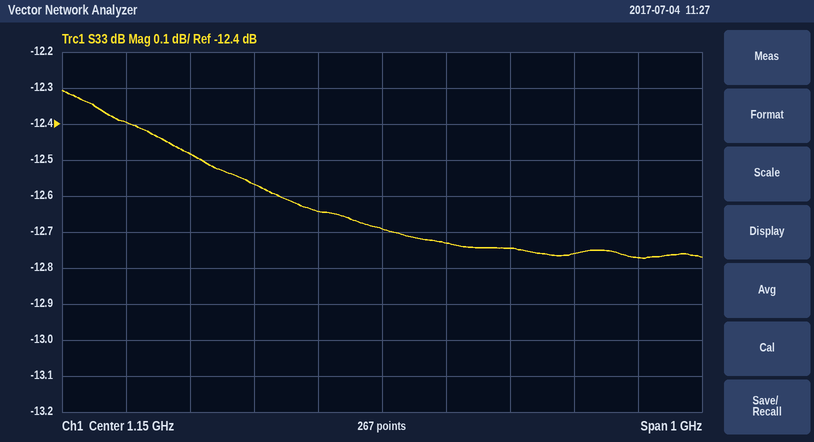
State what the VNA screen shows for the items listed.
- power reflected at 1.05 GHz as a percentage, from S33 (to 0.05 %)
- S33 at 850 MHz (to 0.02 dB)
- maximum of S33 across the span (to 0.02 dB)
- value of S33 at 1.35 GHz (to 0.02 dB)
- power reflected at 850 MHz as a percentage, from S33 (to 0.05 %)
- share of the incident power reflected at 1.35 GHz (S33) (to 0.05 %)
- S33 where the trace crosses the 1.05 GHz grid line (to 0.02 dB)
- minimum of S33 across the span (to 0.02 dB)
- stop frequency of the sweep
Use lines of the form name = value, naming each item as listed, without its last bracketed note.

power reflected at 1.05 GHz as a percentage, from S33 = 5.45 %
S33 at 850 MHz = -12.48 dB
maximum of S33 across the span = -12.30 dB
value of S33 at 1.35 GHz = -12.74 dB
power reflected at 850 MHz as a percentage, from S33 = 5.65 %
share of the incident power reflected at 1.35 GHz (S33) = 5.30 %
S33 where the trace crosses the 1.05 GHz grid line = -12.64 dB
minimum of S33 across the span = -12.78 dB
stop frequency of the sweep = 1.65 GHz
